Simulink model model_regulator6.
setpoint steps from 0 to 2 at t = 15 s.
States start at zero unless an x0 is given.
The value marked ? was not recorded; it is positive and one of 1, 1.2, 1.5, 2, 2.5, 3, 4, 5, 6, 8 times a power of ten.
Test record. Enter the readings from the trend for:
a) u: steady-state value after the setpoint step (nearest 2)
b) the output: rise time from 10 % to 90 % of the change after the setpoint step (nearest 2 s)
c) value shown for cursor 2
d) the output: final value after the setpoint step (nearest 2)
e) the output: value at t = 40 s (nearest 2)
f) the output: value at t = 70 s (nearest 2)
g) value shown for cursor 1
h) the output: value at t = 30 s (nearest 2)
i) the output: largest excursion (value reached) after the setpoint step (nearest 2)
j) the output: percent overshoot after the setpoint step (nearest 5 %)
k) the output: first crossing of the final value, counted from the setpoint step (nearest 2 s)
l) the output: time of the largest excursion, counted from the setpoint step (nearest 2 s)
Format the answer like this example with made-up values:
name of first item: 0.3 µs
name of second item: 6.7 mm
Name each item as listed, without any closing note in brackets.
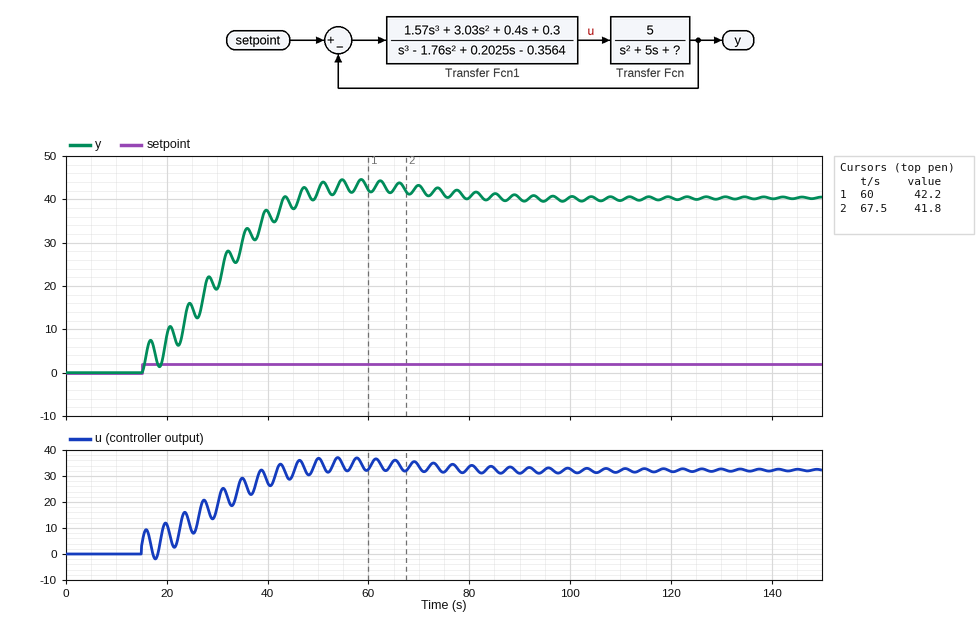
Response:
u: steady-state value after the setpoint step: 32
the output: rise time from 10 % to 90 % of the change after the setpoint step: 24 s
value shown for cursor 2: 41.8
the output: final value after the setpoint step: 40
the output: value at t = 40 s: 38
the output: value at t = 70 s: 44
value shown for cursor 1: 42.2
the output: value at t = 30 s: 20
the output: largest excursion (value reached) after the setpoint step: 44
the output: percent overshoot after the setpoint step: 10 %
the output: first crossing of the final value, counted from the setpoint step: 28 s
the output: time of the largest excursion, counted from the setpoint step: 44 s
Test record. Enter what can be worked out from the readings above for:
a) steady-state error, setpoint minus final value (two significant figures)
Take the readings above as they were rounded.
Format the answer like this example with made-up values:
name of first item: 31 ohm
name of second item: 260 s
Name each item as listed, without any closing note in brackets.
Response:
steady-state error, setpoint minus final value: -38
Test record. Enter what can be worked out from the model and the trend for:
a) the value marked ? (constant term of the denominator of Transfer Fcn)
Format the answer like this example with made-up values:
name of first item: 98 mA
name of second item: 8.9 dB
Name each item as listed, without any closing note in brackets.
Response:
the value marked ?: 4
